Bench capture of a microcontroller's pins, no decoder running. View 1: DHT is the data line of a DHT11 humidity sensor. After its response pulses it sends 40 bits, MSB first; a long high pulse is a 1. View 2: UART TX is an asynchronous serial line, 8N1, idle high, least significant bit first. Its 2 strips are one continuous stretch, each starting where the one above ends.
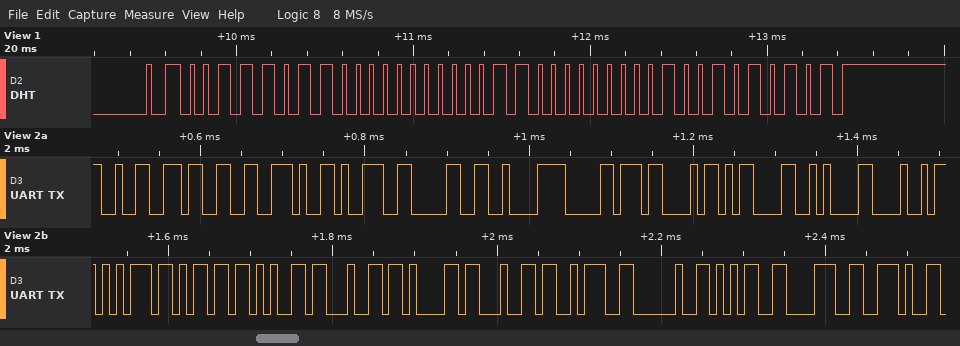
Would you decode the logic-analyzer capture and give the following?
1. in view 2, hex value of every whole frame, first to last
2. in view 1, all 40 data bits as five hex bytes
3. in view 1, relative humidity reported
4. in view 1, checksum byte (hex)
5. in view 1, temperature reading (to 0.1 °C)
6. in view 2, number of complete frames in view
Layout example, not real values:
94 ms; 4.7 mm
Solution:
32 33 2E 39 30 C2 B0 43 0D 0A 48 75 6D 65 64 61 64 3A 20 35 38 2E; 3B 00 18 02 55; 59 %; 0x55; 24.2 °C; 22
